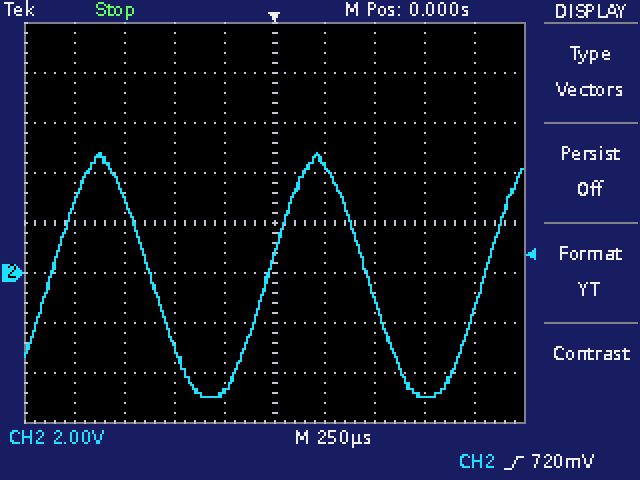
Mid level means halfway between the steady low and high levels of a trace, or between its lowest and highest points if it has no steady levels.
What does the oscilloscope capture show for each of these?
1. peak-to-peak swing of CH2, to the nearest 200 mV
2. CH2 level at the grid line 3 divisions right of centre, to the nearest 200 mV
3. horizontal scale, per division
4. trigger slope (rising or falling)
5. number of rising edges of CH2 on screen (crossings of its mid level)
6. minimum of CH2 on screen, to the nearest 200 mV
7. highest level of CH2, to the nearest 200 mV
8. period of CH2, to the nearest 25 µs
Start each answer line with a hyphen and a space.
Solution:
- 9.8 V
- -5.0 V
- 250 µs
- rising
- 3
- -5.0 V
- 4.8 V
- 1.075 ms
